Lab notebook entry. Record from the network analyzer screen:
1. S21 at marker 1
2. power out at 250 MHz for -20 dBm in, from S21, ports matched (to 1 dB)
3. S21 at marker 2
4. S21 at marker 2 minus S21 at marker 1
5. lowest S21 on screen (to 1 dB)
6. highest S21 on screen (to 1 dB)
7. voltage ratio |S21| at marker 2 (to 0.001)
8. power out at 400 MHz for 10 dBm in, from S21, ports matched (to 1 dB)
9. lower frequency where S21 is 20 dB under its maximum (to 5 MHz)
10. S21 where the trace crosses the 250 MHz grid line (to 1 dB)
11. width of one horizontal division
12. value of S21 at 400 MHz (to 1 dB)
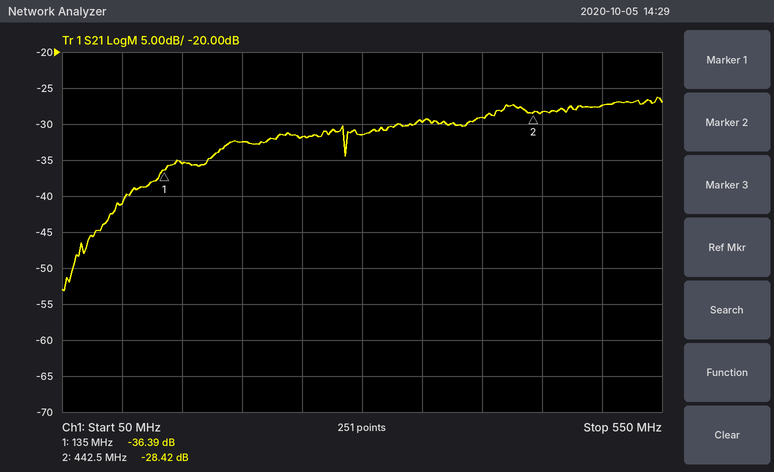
-36.39 dB
-52 dBm
-28.42 dB
7.97 dB
-53 dB
-26 dB
0.038
-19 dBm
70 MHz
-32 dB
50 MHz
-29 dB
